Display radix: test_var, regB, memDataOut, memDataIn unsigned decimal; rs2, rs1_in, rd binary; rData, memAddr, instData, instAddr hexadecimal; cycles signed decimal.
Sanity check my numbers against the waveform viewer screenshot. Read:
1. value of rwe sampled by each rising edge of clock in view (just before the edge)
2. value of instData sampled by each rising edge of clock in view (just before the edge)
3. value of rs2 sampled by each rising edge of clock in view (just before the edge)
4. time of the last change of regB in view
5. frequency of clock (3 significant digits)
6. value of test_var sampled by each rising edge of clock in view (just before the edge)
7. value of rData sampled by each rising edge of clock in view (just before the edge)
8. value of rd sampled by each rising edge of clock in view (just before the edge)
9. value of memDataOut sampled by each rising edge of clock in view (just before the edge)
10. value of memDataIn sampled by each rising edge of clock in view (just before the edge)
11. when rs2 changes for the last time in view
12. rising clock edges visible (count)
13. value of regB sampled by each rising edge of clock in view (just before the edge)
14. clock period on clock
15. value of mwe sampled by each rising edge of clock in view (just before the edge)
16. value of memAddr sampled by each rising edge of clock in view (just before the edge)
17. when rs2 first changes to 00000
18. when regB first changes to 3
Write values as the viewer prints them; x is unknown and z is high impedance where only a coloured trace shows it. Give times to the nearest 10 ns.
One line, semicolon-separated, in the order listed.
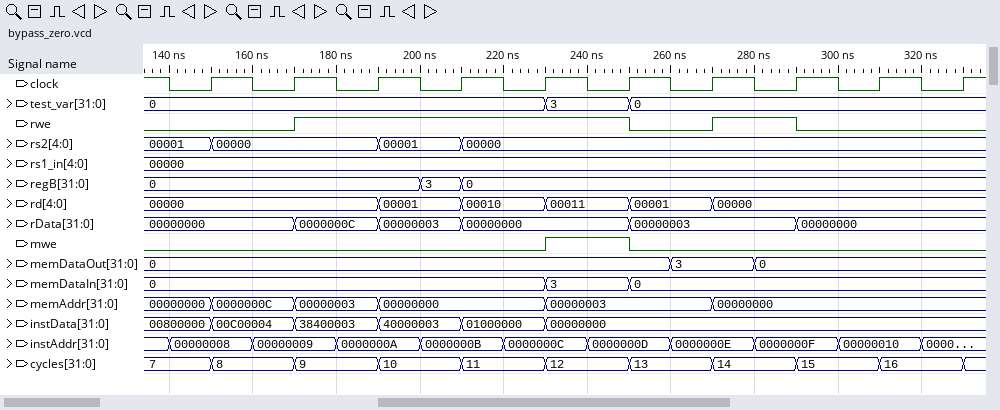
0 0 1 1 1 1 0 1 0 0; 00800000, 00C00004, 38400003, 40000003, 01000000, 00000000, 00000000, 00000000, 00000000, 00000000; 00001, 00000, 00000, 00001, 00000, 00000, 00000, 00000, 00000, 00000; 210 ns; 50.0 MHz; 0, 0, 0, 0, 0, 3, 0, 0, 0, 0; 00000000, 00000000, 0000000C, 00000003, 00000000, 00000000, 00000003, 00000003, 00000000, 00000000; 00000, 00000, 00000, 00001, 00010, 00011, 00001, 00000, 00000, 00000; 0, 0, 0, 0, 0, 0, 3, 0, 0, 0; 0, 0, 0, 0, 0, 3, 0, 0, 0, 0; 210 ns; 10; 0, 0, 0, 3, 0, 0, 0, 0, 0, 0; 20 ns; 0 0 0 0 0 1 0 0 0 0; 00000000, 0000000C, 00000003, 00000000, 00000000, 00000003, 00000003, 00000000, 00000000, 00000000; 150 ns; 200 ns
